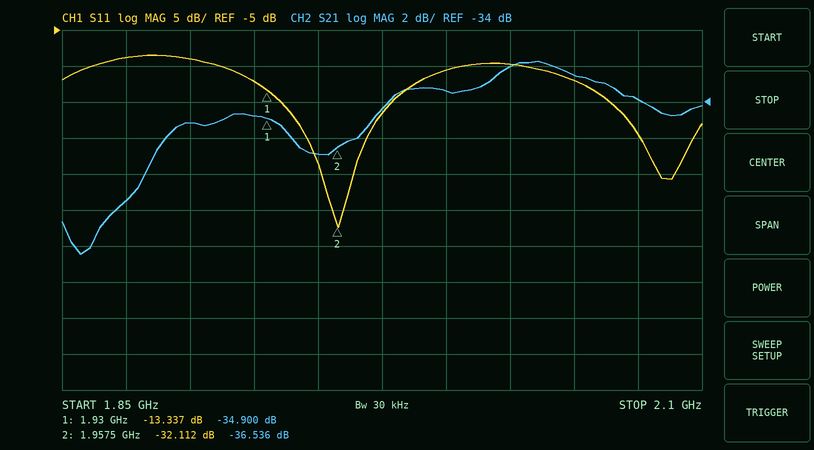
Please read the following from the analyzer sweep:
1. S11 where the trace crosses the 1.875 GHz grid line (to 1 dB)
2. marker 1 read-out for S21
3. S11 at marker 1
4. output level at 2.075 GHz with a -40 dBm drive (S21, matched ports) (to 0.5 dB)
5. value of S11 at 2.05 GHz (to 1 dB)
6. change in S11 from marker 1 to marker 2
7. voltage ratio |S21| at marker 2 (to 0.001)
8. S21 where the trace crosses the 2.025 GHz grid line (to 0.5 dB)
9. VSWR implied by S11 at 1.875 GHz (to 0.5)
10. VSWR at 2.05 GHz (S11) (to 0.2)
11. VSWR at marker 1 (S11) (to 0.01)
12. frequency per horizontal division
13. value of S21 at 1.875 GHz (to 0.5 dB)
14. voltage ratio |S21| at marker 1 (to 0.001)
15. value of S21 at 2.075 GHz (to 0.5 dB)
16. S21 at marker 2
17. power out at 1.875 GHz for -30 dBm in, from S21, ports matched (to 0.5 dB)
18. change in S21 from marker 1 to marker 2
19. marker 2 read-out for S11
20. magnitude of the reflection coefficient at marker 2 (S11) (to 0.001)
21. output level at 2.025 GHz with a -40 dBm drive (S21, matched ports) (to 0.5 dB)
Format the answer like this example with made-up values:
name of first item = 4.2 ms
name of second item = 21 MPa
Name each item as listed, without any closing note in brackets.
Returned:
S11 where the trace crosses the 1.875 GHz grid line = -9 dB
marker 1 read-out for S21 = -34.900 dB
S11 at marker 1 = -13.337 dB
output level at 2.075 GHz with a -40 dBm drive (S21, matched ports) = -74.0 dBm
value of S11 at 2.05 GHz = -12 dB
change in S11 from marker 1 to marker 2 = -18.775 dB
voltage ratio |S21| at marker 2 = 0.015
S21 where the trace crosses the 2.025 GHz grid line = -32.0 dB
VSWR implied by S11 at 1.875 GHz = 2.0
VSWR at 2.05 GHz (S11) = 1.6
VSWR at marker 1 (S11) = 1.55
frequency per horizontal division = 25 MHz
value of S21 at 1.875 GHz = -39.5 dB
voltage ratio |S21| at marker 1 = 0.018
value of S21 at 2.075 GHz = -34.0 dB
S21 at marker 2 = -36.536 dB
power out at 1.875 GHz for -30 dBm in, from S21, ports matched = -69.5 dBm
change in S21 from marker 1 to marker 2 = -1.636 dB
marker 2 read-out for S11 = -32.112 dB
magnitude of the reflection coefficient at marker 2 (S11) = 0.025
output level at 2.025 GHz with a -40 dBm drive (S21, matched ports) = -72.0 dBm
